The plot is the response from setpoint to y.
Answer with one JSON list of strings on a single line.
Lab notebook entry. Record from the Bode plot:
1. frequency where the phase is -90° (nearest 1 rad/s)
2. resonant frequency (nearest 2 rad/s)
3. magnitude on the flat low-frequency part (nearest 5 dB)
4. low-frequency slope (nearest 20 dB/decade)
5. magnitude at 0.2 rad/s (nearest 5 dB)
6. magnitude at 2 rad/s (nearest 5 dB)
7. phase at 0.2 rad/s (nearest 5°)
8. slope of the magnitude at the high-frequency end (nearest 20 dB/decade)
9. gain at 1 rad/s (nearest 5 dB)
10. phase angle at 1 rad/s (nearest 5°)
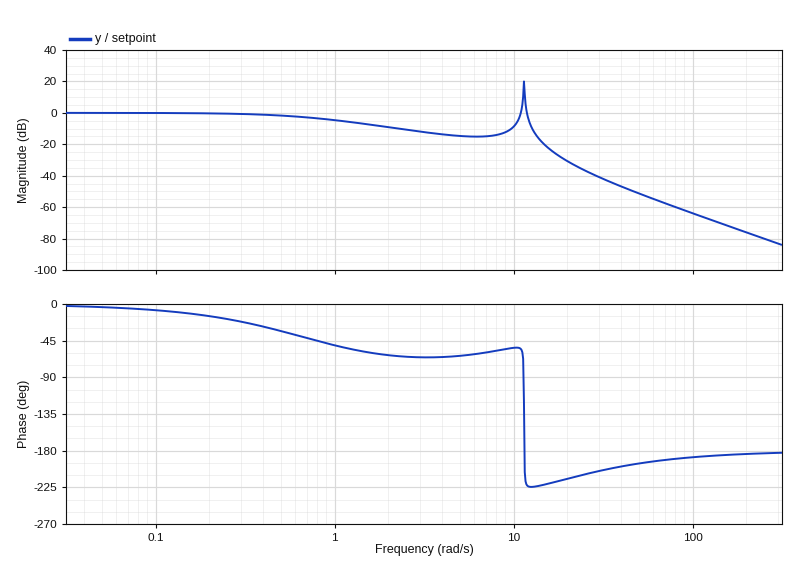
["11 rad/s", "12 rad/s", "0 dB", "0 dB/decade", "0 dB", "-10 dB", "-15°", "-40 dB/decade", "-5 dB", "-50°"]
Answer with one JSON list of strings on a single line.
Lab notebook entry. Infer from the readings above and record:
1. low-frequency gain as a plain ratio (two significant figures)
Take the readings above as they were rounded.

["1.0"]
